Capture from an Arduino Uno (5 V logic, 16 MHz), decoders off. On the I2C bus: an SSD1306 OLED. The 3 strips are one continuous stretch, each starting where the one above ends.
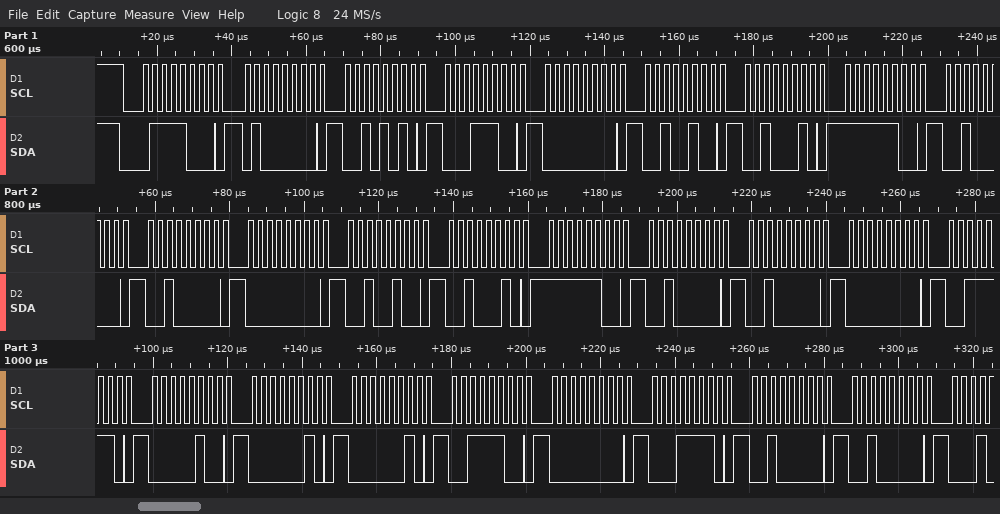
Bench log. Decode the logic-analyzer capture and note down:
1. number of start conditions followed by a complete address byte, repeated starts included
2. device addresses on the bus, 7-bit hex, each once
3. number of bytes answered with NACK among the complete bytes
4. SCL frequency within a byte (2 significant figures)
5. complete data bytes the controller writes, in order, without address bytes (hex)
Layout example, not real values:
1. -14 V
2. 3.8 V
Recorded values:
1. 1
2. 0x3C
3. 0
4. 400 kHz
5. 40 2A 1C 00 24 22 FC 20 20 00 24 22 FC 20 20 00 3E 04 02 02 3C 00 1E 20 20
